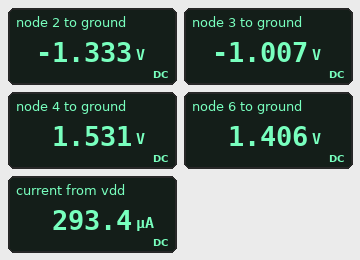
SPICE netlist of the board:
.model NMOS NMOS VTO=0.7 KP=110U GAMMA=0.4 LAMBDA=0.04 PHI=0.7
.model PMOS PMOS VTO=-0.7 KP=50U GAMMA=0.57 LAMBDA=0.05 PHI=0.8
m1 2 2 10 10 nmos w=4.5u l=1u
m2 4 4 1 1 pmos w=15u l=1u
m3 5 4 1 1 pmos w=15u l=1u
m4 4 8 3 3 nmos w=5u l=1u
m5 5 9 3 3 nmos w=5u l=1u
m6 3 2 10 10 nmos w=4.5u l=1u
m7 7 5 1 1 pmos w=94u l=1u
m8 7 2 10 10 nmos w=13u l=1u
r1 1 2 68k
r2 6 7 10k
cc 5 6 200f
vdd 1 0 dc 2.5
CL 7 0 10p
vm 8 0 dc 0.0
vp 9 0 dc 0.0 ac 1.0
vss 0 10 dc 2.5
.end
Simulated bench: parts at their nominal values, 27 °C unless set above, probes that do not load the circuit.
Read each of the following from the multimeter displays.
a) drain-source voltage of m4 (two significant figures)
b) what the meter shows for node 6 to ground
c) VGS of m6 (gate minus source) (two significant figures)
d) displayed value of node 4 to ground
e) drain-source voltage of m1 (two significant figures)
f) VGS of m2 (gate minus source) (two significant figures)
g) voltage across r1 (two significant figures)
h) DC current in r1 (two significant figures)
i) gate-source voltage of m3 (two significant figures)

2.5 V
1.406 V
1.2 V
1.531 V
1.2 V
-970 mV
3.8 V
56 µA
-970 mV
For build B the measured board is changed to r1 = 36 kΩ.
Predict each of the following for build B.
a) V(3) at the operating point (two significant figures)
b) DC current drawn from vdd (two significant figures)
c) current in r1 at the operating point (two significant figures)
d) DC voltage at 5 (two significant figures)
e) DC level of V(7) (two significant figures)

-1.1 V
530 µA
100 µA
1.4 V
1.3 V
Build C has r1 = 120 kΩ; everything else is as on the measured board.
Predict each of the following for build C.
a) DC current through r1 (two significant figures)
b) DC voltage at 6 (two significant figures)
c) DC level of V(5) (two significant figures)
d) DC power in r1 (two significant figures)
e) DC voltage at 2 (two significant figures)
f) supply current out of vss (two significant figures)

33 µA
1.5 V
1.6 V
130 µW
-1.4 V
170 µA
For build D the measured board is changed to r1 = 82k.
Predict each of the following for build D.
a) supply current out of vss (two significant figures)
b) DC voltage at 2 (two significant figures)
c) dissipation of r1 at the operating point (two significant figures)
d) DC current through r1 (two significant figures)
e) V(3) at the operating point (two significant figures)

250 µA
-1.4 V
180 µW
47 µA
-980 mV
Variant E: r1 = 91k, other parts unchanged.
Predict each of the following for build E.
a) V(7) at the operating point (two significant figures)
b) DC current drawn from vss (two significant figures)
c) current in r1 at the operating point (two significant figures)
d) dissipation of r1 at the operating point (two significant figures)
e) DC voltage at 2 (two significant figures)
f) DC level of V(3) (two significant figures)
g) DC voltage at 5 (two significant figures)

1.4 V
220 µA
43 µA
170 µW
-1.4 V
-970 mV
1.6 V
